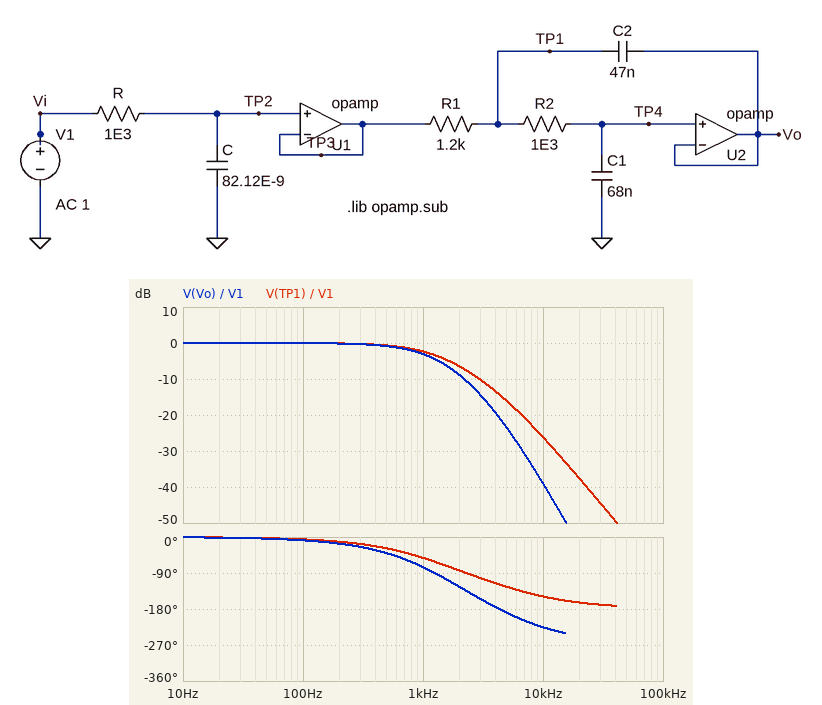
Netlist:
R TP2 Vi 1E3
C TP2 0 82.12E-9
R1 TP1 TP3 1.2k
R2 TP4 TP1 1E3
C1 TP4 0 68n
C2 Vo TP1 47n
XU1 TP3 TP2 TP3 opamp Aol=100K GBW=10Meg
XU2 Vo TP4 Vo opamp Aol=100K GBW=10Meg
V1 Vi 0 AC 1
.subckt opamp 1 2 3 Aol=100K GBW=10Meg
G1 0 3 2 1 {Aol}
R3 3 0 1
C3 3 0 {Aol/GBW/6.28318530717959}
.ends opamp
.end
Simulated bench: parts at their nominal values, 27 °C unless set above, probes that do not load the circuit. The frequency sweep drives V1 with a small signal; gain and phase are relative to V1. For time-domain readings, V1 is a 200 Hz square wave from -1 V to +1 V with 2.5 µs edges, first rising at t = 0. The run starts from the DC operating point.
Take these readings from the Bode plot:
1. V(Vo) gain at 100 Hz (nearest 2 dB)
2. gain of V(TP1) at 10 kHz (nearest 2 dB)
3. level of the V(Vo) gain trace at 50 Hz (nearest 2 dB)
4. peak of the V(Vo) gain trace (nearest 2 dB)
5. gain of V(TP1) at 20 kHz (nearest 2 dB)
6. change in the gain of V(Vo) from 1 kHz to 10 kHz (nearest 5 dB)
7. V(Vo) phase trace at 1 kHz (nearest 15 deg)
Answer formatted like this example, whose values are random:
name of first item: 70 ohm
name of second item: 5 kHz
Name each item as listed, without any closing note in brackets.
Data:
V(Vo) gain at 100 Hz: 0 dB
gain of V(TP1) at 10 kHz: -26 dB
level of the V(Vo) gain trace at 50 Hz: 0 dB
peak of the V(Vo) gain trace: 0 dB
gain of V(TP1) at 20 kHz: -38 dB
change in the gain of V(Vo) from 1 kHz to 10 kHz: -35 dB
V(Vo) phase trace at 1 kHz: -75 deg
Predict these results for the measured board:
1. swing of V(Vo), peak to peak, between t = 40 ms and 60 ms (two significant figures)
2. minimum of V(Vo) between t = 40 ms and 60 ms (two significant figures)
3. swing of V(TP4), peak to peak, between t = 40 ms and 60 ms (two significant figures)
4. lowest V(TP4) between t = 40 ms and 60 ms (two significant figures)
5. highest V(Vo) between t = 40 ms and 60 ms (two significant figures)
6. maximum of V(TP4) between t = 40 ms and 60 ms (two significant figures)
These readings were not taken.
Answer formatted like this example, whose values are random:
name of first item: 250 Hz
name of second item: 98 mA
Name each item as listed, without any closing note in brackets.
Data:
swing of V(Vo), peak to peak, between t = 40 ms and 60 ms: 2.0 V
minimum of V(Vo) between t = 40 ms and 60 ms: -1.0 V
swing of V(TP4), peak to peak, between t = 40 ms and 60 ms: 2.0 V
lowest V(TP4) between t = 40 ms and 60 ms: -1.0 V
highest V(Vo) between t = 40 ms and 60 ms: 1.0 V
maximum of V(TP4) between t = 40 ms and 60 ms: 1.0 V
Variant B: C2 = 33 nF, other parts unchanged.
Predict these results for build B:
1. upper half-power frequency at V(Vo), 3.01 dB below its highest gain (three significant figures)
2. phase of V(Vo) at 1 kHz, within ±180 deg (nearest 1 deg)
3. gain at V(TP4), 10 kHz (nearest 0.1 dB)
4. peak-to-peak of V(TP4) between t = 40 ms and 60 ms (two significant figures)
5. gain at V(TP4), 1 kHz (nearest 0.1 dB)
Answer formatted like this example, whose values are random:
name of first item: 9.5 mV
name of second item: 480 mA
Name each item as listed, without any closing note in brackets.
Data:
upper half-power frequency at V(Vo), 3.01 dB below its highest gain: 949 Hz
phase of V(Vo) at 1 kHz, within ±180 deg: -74 deg
gain at V(TP4), 10 kHz: -37.0 dB
peak-to-peak of V(TP4) between t = 40 ms and 60 ms: 2.0 V
gain at V(TP4), 1 kHz: -3.3 dB
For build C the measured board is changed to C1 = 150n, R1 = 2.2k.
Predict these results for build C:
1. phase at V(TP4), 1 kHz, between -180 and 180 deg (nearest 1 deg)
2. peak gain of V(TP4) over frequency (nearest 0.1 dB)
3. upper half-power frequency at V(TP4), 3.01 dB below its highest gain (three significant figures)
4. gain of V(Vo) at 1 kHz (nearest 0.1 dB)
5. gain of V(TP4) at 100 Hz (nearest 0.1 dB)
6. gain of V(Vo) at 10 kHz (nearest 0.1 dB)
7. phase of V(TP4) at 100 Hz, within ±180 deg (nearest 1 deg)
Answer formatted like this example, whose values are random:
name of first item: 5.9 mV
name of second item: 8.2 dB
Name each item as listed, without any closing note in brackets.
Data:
phase at V(TP4), 1 kHz, between -180 and 180 deg: -110 deg
peak gain of V(TP4) over frequency: 0 dB
upper half-power frequency at V(TP4), 3.01 dB below its highest gain: 344 Hz
gain of V(Vo) at 1 kHz: -10.7 dB
gain of V(TP4) at 100 Hz: -0.3 dB
gain of V(Vo) at 10 kHz: -51.0 dB
phase of V(TP4) at 100 Hz, within ±180 deg: -20 deg
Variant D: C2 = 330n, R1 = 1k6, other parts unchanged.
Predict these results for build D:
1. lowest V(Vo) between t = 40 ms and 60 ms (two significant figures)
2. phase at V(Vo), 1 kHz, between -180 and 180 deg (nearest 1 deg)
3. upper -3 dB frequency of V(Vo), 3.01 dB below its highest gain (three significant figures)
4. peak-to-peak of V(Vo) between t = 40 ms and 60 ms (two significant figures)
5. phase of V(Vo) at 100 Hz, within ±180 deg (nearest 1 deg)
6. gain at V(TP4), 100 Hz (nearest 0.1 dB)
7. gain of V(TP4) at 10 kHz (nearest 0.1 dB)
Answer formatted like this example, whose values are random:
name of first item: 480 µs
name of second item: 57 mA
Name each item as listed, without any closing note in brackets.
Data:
lowest V(Vo) between t = 40 ms and 60 ms: -1.3 V
phase at V(Vo), 1 kHz, between -180 and 180 deg: -138 deg
upper -3 dB frequency of V(Vo), 3.01 dB below its highest gain: 954 Hz
peak-to-peak of V(Vo) between t = 40 ms and 60 ms: 2.7 V
phase of V(Vo) at 100 Hz, within ±180 deg: -9 deg
gain at V(TP4), 100 Hz: 0.1 dB
gain of V(TP4) at 10 kHz: -57.4 dB
